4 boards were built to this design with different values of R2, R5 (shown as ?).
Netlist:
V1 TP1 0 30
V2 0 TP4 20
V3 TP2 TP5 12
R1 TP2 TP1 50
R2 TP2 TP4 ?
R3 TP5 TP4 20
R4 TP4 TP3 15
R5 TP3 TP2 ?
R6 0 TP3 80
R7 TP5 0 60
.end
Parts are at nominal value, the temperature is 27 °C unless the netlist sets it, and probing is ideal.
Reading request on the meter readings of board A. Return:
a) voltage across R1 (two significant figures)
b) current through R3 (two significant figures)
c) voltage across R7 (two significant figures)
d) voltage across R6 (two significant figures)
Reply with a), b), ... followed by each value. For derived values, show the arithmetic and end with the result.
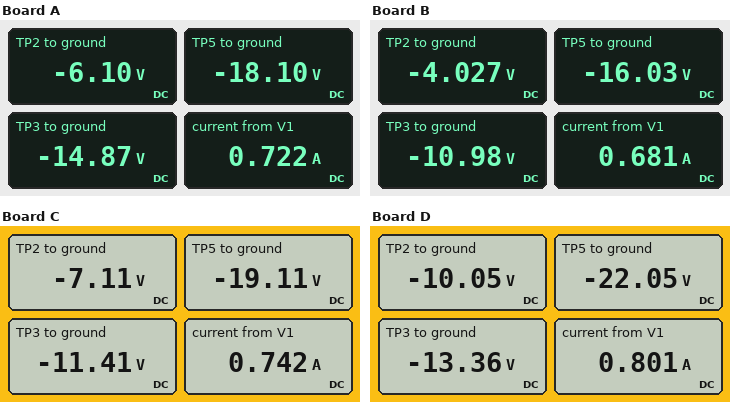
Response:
a) 30 V - (-6.1 V) = 36 V
b) (-18.1 V - (-20 V)) / 20 Ω = 95 mA
c) 0 V - (-18.1 V) = 18 V
d) 0 V - (-14.87 V) = 15 V
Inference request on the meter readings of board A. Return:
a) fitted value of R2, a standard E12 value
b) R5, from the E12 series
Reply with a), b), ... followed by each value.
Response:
a) 18 Ω
b) 56 Ω
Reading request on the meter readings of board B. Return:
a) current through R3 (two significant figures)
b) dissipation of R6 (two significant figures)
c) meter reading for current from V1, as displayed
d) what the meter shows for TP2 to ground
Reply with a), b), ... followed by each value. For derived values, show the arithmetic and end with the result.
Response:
a) (-16.03 V - (-20 V)) / 20 Ω = 200 mA
b) (0 V - (-10.98 V))^2 / 80 Ω = 1.5 W
c) 0.681 A
d) -4.027 V
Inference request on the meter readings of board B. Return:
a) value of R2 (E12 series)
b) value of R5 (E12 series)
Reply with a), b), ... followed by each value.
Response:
a) 56 Ω
b) 15 Ω
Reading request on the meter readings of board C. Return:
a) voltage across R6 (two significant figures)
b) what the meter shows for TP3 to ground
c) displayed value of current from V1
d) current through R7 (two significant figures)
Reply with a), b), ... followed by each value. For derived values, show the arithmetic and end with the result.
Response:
a) 0 V - (-11.41 V) = 11 V
b) -11.41 V
c) 0.742 A
d) (0 V - (-19.11 V)) / 60 Ω = 320 mA
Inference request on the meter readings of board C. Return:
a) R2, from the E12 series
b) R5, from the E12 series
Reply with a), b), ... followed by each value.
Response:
a) 22 Ω
b) 10 Ω
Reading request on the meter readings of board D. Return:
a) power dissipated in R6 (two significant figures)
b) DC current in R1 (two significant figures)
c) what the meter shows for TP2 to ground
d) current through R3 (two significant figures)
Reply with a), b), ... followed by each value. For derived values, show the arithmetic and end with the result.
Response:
a) (0 V - (-13.36 V))^2 / 80 Ω = 2.2 W
b) (30 V - (-10.05 V)) / 50 Ω = 800 mA
c) -10.05 V
d) (-20 V - (-22.05 V)) / 20 Ω = 100 mA
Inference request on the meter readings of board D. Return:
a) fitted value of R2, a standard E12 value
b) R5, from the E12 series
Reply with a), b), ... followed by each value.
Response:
a) 10 Ω
b) 12 Ω
